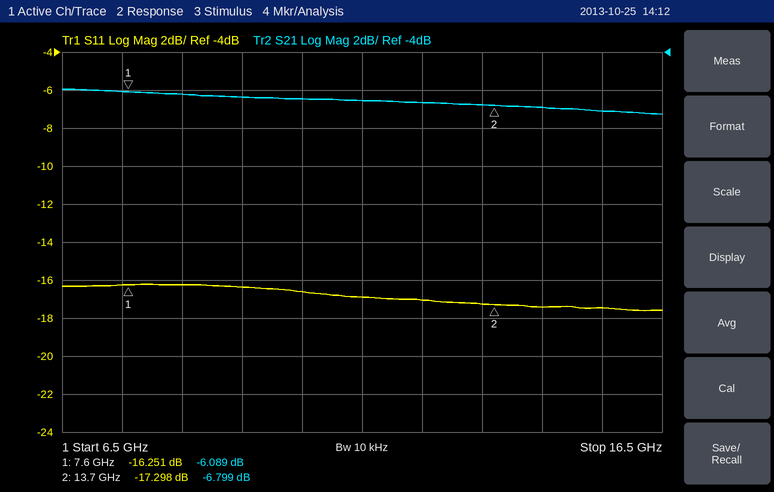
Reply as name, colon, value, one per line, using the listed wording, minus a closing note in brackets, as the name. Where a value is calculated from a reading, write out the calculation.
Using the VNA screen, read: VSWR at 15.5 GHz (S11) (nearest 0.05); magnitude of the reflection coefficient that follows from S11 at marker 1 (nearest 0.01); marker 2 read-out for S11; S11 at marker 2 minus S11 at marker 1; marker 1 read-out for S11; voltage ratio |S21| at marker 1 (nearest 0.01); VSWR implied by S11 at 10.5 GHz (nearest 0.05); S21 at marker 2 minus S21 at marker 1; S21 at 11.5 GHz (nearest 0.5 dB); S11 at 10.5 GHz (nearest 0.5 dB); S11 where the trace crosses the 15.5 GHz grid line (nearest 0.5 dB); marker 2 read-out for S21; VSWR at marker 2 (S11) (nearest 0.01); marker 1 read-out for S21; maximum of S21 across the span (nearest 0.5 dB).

VSWR at 15.5 GHz (S11): |Γ| = 10^(-17.5/20) = 0.1334; VSWR = (1 + 0.1334)/(1 − 0.1334) ≈ 1.31, so 1.30 to the nearest 0.05
magnitude of the reflection coefficient that follows from S11 at marker 1: 10^(-16.251/20) ≈ 0.15
marker 2 read-out for S11: -17.298 dB
S11 at marker 2 minus S11 at marker 1: -17.298 − (-16.251) = -1.047 dB
marker 1 read-out for S11: -16.251 dB
voltage ratio |S21| at marker 1: 10^(-6.089/20) ≈ 0.50
VSWR implied by S11 at 10.5 GHz: |Γ| = 10^(-16.5/20) = 0.1496; VSWR = (1 + 0.1496)/(1 − 0.1496) ≈ 1.35
S21 at marker 2 minus S21 at marker 1: -6.799 − (-6.089) = -0.710 dB
S21 at 11.5 GHz: -6.5 dB
S11 at 10.5 GHz: -16.5 dB
S11 where the trace crosses the 15.5 GHz grid line: -17.5 dB
marker 2 read-out for S21: -6.799 dB
VSWR at marker 2 (S11): (1 + 0.1365)/(1 − 0.1365) ≈ 1.32
marker 1 read-out for S21: -6.089 dB
maximum of S21 across the span: -6.0 dB
